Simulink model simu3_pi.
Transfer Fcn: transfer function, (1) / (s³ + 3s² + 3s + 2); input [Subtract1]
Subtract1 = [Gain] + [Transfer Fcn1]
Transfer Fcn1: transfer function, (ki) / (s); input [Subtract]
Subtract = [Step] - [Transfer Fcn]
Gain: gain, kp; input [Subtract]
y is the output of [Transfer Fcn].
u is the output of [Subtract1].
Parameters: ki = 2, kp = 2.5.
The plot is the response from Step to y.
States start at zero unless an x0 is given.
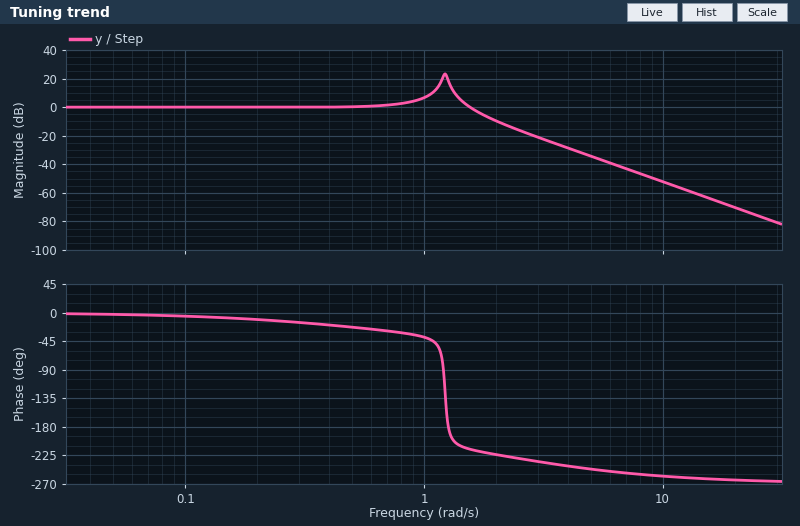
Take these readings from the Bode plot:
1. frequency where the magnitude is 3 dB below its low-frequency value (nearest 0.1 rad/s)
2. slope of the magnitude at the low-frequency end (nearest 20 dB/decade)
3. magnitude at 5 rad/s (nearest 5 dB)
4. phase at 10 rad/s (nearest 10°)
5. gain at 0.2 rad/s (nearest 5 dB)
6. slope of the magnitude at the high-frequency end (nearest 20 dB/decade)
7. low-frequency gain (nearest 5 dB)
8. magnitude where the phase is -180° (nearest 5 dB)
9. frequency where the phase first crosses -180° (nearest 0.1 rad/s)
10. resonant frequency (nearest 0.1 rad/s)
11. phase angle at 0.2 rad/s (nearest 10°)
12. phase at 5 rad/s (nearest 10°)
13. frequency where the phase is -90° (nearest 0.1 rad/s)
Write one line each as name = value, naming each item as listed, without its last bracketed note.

frequency where the magnitude is 3 dB below its low-frequency value = 1.7 rad/s
slope of the magnitude at the low-frequency end = 0 dB/decade
magnitude at 5 rad/s = -35 dB
phase at 10 rad/s = -260°
gain at 0.2 rad/s = 0 dB
slope of the magnitude at the high-frequency end = -60 dB/decade
low-frequency gain = 0 dB
magnitude where the phase is -180° = 20 dB
frequency where the phase first crosses -180° = 1.3 rad/s
resonant frequency = 1.2 rad/s
phase angle at 0.2 rad/s = -10°
phase at 5 rad/s = -250°
frequency where the phase is -90° = 1.2 rad/s
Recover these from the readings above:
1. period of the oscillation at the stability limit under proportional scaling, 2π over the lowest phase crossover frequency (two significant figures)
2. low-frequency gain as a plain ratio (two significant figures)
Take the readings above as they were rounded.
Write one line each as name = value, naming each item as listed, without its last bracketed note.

period of the oscillation at the stability limit under proportional scaling, 2π over the lowest phase crossover frequency = 4.8 s
low-frequency gain as a plain ratio = 1.0
